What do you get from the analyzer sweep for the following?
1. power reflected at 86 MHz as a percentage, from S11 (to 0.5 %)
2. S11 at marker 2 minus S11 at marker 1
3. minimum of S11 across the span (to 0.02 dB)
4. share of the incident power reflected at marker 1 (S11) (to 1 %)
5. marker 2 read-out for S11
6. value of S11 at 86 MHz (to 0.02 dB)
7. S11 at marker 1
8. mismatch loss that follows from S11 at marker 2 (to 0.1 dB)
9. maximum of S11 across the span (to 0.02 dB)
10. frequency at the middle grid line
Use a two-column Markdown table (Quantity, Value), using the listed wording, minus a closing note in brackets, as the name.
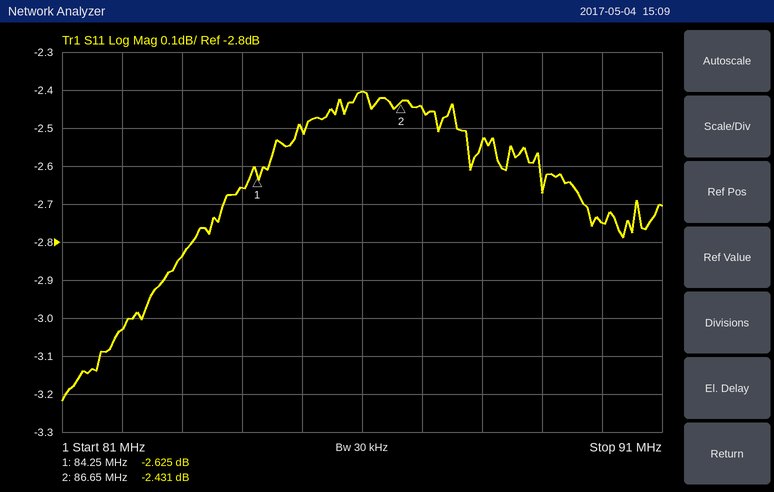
| Quantity | Value |
|---|---|
| power reflected at 86 MHz as a percentage, from S11 | 57.5 % |
| S11 at marker 2 minus S11 at marker 1 | 0.194 dB |
| minimum of S11 across the span | -3.22 dB |
| share of the incident power reflected at marker 1 (S11) | 55 % |
| marker 2 read-out for S11 | -2.431 dB |
| value of S11 at 86 MHz | -2.40 dB |
| S11 at marker 1 | -2.625 dB |
| mismatch loss that follows from S11 at marker 2 | 3.7 dB |
| maximum of S11 across the span | -2.40 dB |
| frequency at the middle grid line | 86 MHz |
